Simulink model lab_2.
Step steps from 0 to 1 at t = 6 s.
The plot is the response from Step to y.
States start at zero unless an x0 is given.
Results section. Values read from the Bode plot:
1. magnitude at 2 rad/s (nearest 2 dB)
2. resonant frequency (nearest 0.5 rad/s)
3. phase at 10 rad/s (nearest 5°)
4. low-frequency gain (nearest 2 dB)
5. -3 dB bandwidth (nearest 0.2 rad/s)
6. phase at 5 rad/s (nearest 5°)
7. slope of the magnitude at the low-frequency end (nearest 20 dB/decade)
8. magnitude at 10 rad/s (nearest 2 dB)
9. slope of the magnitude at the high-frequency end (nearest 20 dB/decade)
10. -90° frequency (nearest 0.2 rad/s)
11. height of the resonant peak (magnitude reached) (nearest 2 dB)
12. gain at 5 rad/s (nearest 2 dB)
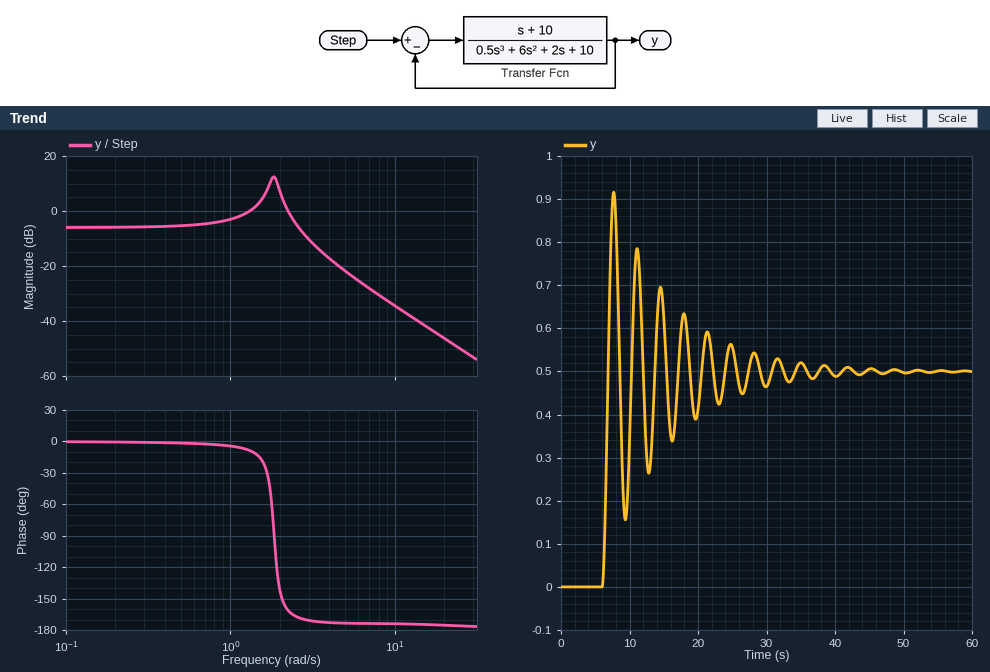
8 dB
2.0 rad/s
-175°
-6 dB
2.8 rad/s
-175°
0 dB/decade
-34 dB
-40 dB/decade
1.8 rad/s
12 dB
-22 dB
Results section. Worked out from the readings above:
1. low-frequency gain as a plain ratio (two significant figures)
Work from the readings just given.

0.50
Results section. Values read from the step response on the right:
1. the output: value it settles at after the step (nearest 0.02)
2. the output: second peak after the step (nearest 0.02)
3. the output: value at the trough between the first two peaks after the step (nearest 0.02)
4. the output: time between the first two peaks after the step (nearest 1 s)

0.50
0.78
0.16
3 s
